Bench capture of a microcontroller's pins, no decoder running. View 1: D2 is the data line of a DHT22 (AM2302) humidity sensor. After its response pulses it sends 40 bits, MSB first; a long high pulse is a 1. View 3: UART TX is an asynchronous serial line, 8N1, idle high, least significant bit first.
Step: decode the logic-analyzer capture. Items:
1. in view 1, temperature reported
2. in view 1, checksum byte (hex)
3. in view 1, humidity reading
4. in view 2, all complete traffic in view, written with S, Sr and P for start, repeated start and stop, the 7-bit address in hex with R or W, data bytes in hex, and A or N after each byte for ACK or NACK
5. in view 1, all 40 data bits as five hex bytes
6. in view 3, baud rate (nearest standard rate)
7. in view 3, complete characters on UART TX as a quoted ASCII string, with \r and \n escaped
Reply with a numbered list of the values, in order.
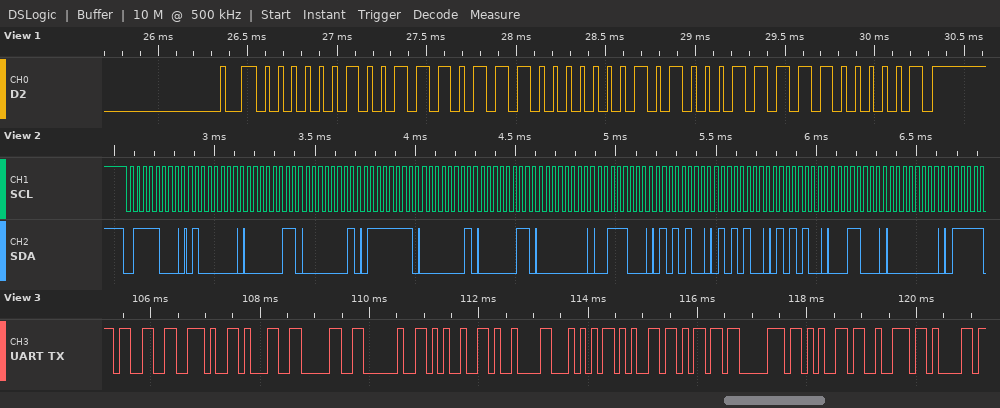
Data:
1. 32.7 °C
2. 0xC1
3. 63.1 %
4. S 3CW A 40 A 03 A 01 A 7F A 01 A 03 A 00 A 38 A 54 A 54 A 54 A 18 A 00 A
5. 02 77 01 47 C1
6. 9600 baud
7. "3.10 %\tTempera"
